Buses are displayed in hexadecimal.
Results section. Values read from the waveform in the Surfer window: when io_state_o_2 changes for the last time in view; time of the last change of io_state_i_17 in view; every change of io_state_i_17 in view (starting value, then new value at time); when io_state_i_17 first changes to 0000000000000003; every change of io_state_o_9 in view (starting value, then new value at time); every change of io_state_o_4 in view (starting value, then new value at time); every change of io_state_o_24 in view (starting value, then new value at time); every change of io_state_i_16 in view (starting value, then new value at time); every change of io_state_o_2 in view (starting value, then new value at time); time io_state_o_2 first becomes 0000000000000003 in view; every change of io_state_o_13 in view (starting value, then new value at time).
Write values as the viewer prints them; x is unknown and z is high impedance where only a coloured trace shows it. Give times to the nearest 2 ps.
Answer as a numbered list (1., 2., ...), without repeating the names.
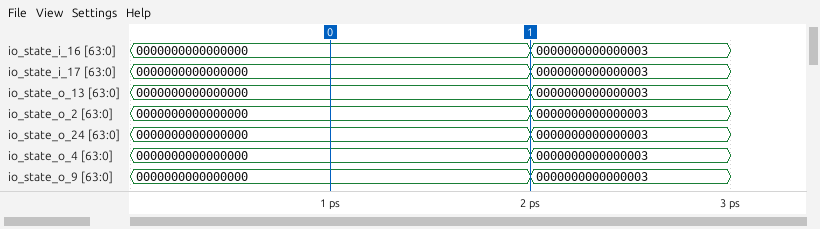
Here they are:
1. 2 ps
2. 2 ps
3. 0000000000000000, 0000000000000003 at 2 ps
4. 2 ps
5. 0000000000000000, 0000000000000003 at 2 ps
6. 0000000000000000, 0000000000000003 at 2 ps
7. 0000000000000000, 0000000000000003 at 2 ps
8. 0000000000000000, 0000000000000003 at 2 ps
9. 0000000000000000, 0000000000000003 at 2 ps
10. 2 ps
11. 0000000000000000, 0000000000000003 at 2 ps
